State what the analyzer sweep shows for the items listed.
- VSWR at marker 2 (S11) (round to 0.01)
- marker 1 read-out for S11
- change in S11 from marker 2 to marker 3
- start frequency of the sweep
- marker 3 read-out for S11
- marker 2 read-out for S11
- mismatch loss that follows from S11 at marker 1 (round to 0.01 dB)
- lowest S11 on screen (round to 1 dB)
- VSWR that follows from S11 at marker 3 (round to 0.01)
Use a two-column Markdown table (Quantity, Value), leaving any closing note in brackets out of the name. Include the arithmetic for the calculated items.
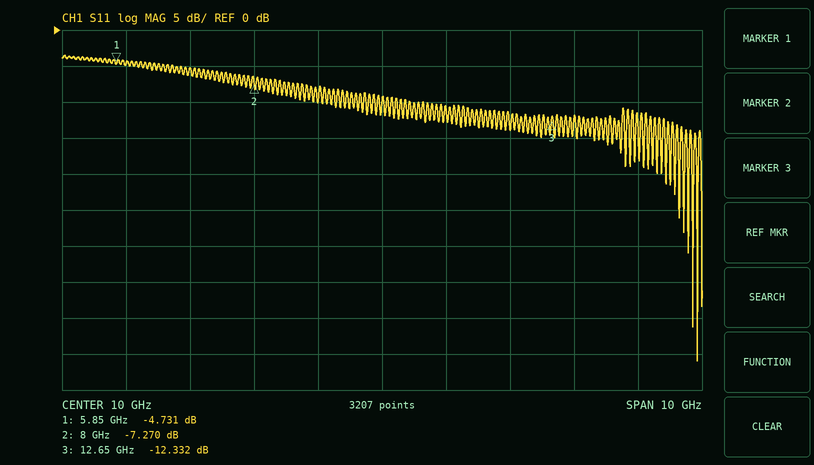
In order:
| Quantity | Value |
|---|---|
| VSWR at marker 2 (S11) | (1 + 0.4330)/(1 − 0.4330) ≈ 2.53 |
| marker 1 read-out for S11 | -4.731 dB |
| change in S11 from marker 2 to marker 3 | -12.332 − (-7.27) = -5.062 dB |
| start frequency of the sweep | 5 GHz |
| marker 3 read-out for S11 | -12.332 dB |
| marker 2 read-out for S11 | -7.270 dB |
| mismatch loss that follows from S11 at marker 1 | −10 log10(1 − 10^(-4.731/10)) ≈ 1.78 dB |
| lowest S11 on screen | -46 dB |
| VSWR that follows from S11 at marker 3 | (1 + 0.2418)/(1 − 0.2418) ≈ 1.64 |
